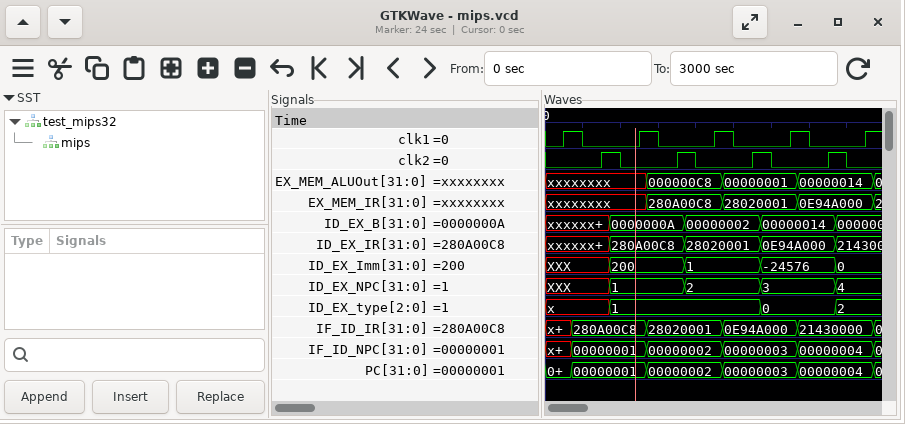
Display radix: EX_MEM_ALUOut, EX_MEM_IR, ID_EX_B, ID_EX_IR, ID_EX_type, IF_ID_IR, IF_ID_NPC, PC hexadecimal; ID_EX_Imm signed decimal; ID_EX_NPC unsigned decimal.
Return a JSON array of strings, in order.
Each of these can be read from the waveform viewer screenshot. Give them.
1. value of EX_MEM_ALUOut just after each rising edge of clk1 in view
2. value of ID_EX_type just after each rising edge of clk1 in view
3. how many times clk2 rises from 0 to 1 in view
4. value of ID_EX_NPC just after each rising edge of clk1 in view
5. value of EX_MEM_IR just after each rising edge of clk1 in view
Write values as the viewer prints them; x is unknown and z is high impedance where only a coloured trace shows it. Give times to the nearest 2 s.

["xxxxxxxx, xxxxxxxx, 000000C8, 00000001, 00000014", "x, 1, 1, 0, 2", "4", "XXX, 1, 2, 3, 4", "xxxxxxxx, xxxxxxxx, 280A00C8, 28020001, 0E94A000"]
